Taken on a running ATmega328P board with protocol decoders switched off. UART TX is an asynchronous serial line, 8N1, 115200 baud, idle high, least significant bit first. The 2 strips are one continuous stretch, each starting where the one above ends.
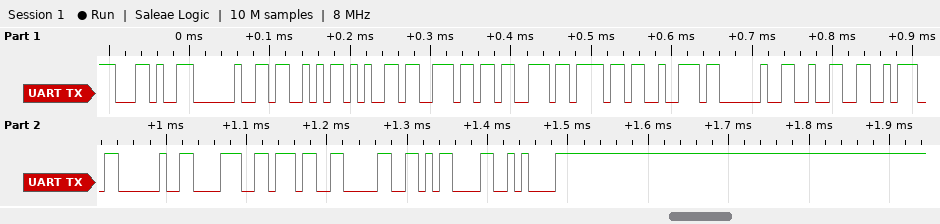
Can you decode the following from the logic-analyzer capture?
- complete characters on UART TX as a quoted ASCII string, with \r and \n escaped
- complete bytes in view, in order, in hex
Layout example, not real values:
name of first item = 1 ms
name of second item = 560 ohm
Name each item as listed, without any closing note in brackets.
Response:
complete characters on UART TX as a quoted ASCII string, with \r and \n escaped = ", Sensor 2: 870\r\n"
complete bytes in view, in order, in hex = 2C 20 53 65 6E 73 6F 72 20 32 3A 20 38 37 30 0D 0A
